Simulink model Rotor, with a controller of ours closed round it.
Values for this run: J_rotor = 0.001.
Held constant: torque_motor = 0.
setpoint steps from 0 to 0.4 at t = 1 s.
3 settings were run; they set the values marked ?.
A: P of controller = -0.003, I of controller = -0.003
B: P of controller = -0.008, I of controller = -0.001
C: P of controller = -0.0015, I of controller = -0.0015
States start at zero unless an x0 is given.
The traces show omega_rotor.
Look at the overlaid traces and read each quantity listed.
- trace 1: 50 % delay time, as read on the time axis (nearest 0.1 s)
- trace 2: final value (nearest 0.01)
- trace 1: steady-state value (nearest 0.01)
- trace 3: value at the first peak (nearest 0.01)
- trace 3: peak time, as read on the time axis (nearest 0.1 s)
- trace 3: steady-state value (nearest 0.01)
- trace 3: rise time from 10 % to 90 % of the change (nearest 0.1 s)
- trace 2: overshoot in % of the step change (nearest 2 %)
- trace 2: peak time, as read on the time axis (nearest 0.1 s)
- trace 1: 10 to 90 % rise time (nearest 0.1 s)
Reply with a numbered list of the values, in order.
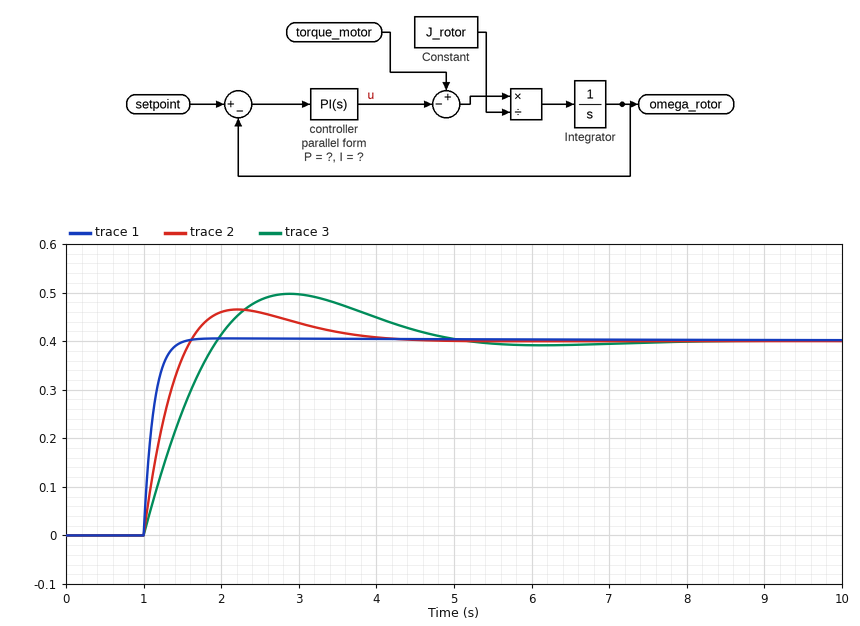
1. 1.1 s
2. 0.40
3. 0.40
4. 0.50
5. 2.9 s
6. 0.40
7. 0.7 s
8. 16 %
9. 2.2 s
10. 0.3 s
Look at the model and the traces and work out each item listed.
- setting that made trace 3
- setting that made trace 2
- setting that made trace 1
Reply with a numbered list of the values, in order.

1. C
2. A
3. B
